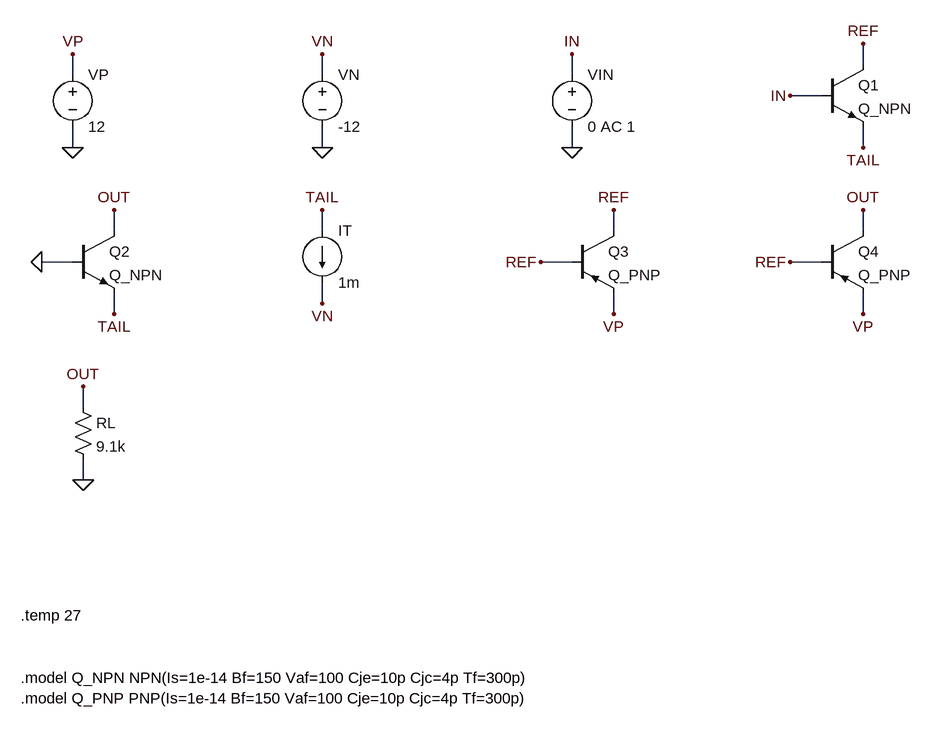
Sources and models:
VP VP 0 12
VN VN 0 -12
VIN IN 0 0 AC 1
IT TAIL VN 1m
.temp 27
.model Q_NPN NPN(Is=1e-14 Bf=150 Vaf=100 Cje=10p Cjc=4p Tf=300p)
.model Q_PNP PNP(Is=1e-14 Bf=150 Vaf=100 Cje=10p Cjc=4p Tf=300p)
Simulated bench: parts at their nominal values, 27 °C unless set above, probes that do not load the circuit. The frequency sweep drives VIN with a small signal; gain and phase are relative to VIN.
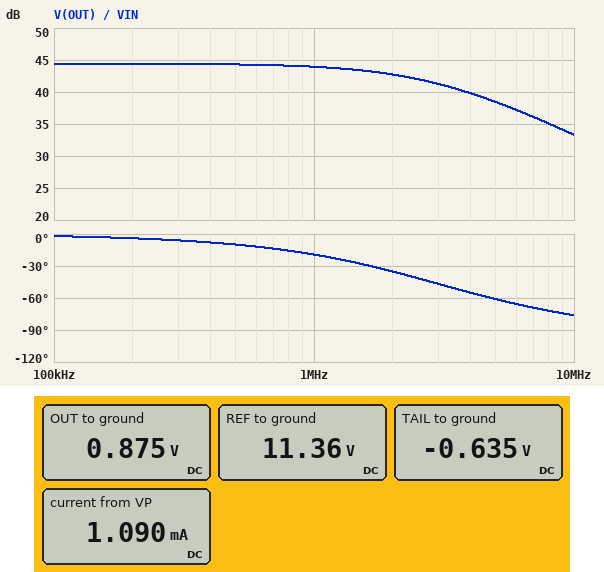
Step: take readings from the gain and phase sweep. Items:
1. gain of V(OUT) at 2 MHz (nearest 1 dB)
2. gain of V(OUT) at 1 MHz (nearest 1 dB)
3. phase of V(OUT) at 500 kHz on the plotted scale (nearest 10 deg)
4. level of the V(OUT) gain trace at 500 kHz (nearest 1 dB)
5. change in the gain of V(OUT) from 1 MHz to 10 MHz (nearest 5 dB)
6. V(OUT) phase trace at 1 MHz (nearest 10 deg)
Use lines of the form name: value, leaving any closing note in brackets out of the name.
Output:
gain of V(OUT) at 2 MHz: 43 dB
gain of V(OUT) at 1 MHz: 44 dB
phase of V(OUT) at 500 kHz on the plotted scale: -10 deg
level of the V(OUT) gain trace at 500 kHz: 44 dB
change in the gain of V(OUT) from 1 MHz to 10 MHz: -10 dB
V(OUT) phase trace at 1 MHz: -20 deg
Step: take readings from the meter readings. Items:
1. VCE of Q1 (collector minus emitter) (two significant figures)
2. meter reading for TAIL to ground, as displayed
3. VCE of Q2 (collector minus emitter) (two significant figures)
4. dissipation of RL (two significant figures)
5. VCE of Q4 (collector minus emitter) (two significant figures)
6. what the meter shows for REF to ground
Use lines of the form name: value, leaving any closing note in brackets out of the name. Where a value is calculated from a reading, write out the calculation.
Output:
VCE of Q1 (collector minus emitter): 11.36 V - (-635 mV) = 12 V
meter reading for TAIL to ground, as displayed: -0.635 V
VCE of Q2 (collector minus emitter): 875 mV - (-635 mV) = 1.5 V
dissipation of RL: (875 mV)^2 / 9.1 kΩ = 84 µW
VCE of Q4 (collector minus emitter): 875 mV - 12 V = -11 V
what the meter shows for REF to ground: 11.36 V
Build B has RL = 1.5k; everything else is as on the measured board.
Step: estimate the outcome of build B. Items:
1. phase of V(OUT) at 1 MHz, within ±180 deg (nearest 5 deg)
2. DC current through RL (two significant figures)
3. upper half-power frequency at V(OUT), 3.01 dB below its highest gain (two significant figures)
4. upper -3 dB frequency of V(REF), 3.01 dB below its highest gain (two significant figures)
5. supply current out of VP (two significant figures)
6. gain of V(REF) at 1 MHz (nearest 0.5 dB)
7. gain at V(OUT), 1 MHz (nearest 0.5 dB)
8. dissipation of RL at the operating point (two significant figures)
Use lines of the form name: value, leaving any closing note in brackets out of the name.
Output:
phase of V(OUT) at 1 MHz, within ±180 deg: -5 deg
DC current through RL: 100 µA
upper half-power frequency at V(OUT), 3.01 dB below its highest gain: 14 MHz
upper -3 dB frequency of V(REF), 3.01 dB below its highest gain: 19 MHz
supply current out of VP: 1.1 mA
gain of V(REF) at 1 MHz: -6.5 dB
gain at V(OUT), 1 MHz: 29.5 dB
dissipation of RL at the operating point: 16 µW
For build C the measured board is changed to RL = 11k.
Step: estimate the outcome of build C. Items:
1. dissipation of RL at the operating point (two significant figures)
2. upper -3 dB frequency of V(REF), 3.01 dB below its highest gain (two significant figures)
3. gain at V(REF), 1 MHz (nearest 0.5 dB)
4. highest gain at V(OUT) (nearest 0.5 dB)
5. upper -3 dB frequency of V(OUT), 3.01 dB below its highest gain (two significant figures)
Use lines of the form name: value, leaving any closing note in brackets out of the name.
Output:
dissipation of RL at the operating point: 98 µW
upper -3 dB frequency of V(REF), 3.01 dB below its highest gain: 3.4 MHz
gain at V(REF), 1 MHz: -7.5 dB
highest gain at V(OUT): 46.0 dB
upper -3 dB frequency of V(OUT), 3.01 dB below its highest gain: 2.5 MHz
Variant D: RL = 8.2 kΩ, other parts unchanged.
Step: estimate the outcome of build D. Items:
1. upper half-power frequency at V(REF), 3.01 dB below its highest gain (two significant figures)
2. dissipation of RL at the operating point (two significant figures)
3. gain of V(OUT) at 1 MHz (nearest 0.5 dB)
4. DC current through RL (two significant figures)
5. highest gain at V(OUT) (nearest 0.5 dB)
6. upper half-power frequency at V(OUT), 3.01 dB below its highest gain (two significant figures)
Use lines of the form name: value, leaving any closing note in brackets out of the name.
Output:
upper half-power frequency at V(REF), 3.01 dB below its highest gain: 4.4 MHz
dissipation of RL at the operating point: 77 µW
gain of V(OUT) at 1 MHz: 43.0 dB
DC current through RL: 97 µA
highest gain at V(OUT): 43.5 dB
upper half-power frequency at V(OUT), 3.01 dB below its highest gain: 3.2 MHz
